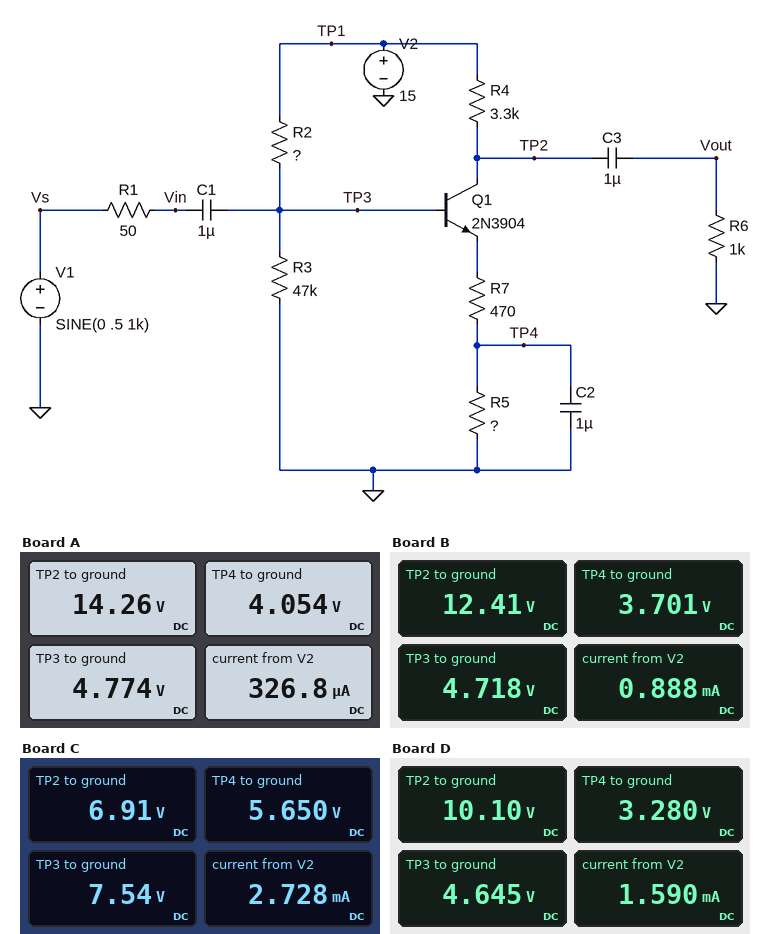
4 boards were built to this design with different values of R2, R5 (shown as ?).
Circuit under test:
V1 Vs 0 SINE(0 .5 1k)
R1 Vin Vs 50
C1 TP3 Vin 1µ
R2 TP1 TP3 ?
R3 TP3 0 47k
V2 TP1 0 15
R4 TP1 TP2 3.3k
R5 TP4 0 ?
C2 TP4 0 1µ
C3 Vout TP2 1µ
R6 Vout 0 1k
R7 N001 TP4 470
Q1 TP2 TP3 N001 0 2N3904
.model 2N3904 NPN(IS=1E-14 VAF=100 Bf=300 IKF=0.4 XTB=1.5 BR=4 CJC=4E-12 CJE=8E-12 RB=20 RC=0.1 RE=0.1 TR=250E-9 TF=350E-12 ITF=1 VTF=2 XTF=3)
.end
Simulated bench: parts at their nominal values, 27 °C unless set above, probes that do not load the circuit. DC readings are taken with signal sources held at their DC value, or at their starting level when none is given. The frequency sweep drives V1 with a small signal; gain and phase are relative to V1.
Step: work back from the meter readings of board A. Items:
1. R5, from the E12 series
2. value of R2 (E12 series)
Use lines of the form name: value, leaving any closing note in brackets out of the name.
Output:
R5, from the E12 series: 18 kΩ
value of R2: 100 kΩ
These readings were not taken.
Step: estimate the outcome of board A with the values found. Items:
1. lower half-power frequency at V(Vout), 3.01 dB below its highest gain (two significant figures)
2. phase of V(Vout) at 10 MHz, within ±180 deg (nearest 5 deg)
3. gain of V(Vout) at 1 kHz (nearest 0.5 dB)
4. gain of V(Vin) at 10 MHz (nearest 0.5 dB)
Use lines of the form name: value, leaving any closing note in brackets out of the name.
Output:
lower half-power frequency at V(Vout), 3.01 dB below its highest gain: 290 Hz
phase of V(Vout) at 10 MHz, within ±180 deg: 165 deg
gain of V(Vout) at 1 kHz: 2.0 dB
gain of V(Vin) at 10 MHz: 0 dB
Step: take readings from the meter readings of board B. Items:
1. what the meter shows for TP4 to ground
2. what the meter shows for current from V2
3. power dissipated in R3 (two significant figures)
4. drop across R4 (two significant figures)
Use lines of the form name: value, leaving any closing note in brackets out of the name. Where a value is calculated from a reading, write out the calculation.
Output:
what the meter shows for TP4 to ground: 3.701 V
what the meter shows for current from V2: 0.888 mA
power dissipated in R3: (4.718 V)^2 / 47 kΩ = 470 µW
drop across R4: 15 V - 12.41 V = 2.6 V
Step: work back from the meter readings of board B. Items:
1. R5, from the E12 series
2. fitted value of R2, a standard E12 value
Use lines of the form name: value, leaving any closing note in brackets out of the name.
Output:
R5, from the E12 series: 4.7 kΩ
fitted value of R2, a standard E12 value: 100 kΩ
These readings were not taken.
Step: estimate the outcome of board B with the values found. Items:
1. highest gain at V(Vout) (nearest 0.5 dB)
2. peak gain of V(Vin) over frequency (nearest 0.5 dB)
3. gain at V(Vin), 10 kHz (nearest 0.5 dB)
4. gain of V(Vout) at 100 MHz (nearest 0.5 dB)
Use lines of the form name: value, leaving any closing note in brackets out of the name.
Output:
highest gain at V(Vout): 3.5 dB
peak gain of V(Vin) over frequency: 0 dB
gain at V(Vin), 10 kHz: 0 dB
gain of V(Vout) at 100 MHz: 2.0 dB
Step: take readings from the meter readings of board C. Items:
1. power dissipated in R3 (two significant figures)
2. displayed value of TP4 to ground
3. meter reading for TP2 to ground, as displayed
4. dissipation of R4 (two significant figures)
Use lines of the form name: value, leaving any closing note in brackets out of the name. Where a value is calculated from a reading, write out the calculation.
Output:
power dissipated in R3: (7.54 V)^2 / 47 kΩ = 1.2 mW
displayed value of TP4 to ground: 5.650 V
meter reading for TP2 to ground, as displayed: 6.91 V
dissipation of R4: (15 V - 6.91 V)^2 / 3.3 kΩ = 20 mW
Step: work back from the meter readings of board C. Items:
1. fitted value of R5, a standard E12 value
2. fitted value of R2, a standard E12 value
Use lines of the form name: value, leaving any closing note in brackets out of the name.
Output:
fitted value of R5, a standard E12 value: 2.2 kΩ
fitted value of R2, a standard E12 value: 27 kΩ
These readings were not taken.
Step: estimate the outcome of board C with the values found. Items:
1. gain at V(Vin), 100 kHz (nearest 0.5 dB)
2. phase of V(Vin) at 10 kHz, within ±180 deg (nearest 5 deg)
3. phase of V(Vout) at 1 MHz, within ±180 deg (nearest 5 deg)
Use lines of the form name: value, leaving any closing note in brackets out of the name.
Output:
gain at V(Vin), 100 kHz: -1.0 dB
phase of V(Vin) at 10 kHz, within ±180 deg: 0 deg
phase of V(Vout) at 1 MHz, within ±180 deg: 5 deg
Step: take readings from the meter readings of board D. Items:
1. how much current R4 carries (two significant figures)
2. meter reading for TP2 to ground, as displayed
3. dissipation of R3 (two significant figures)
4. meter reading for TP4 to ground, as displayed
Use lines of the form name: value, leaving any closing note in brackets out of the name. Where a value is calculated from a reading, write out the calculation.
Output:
how much current R4 carries: (15 V - 10.1 V) / 3.3 kΩ = 1.5 mA
meter reading for TP2 to ground, as displayed: 10.10 V
dissipation of R3: (4.645 V)^2 / 47 kΩ = 460 µW
meter reading for TP4 to ground, as displayed: 3.280 V
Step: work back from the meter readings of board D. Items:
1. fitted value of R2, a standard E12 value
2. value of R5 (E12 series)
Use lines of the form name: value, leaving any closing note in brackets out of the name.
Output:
fitted value of R2, a standard E12 value: 100 kΩ
value of R5: 2.2 kΩ
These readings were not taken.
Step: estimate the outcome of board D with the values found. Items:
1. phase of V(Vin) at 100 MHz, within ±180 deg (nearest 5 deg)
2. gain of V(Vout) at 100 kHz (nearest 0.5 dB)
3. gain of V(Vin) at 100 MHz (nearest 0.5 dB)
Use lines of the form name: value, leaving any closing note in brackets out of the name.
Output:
phase of V(Vin) at 100 MHz, within ±180 deg: -5 deg
gain of V(Vout) at 100 kHz: 4.0 dB
gain of V(Vin) at 100 MHz: -1.0 dB
